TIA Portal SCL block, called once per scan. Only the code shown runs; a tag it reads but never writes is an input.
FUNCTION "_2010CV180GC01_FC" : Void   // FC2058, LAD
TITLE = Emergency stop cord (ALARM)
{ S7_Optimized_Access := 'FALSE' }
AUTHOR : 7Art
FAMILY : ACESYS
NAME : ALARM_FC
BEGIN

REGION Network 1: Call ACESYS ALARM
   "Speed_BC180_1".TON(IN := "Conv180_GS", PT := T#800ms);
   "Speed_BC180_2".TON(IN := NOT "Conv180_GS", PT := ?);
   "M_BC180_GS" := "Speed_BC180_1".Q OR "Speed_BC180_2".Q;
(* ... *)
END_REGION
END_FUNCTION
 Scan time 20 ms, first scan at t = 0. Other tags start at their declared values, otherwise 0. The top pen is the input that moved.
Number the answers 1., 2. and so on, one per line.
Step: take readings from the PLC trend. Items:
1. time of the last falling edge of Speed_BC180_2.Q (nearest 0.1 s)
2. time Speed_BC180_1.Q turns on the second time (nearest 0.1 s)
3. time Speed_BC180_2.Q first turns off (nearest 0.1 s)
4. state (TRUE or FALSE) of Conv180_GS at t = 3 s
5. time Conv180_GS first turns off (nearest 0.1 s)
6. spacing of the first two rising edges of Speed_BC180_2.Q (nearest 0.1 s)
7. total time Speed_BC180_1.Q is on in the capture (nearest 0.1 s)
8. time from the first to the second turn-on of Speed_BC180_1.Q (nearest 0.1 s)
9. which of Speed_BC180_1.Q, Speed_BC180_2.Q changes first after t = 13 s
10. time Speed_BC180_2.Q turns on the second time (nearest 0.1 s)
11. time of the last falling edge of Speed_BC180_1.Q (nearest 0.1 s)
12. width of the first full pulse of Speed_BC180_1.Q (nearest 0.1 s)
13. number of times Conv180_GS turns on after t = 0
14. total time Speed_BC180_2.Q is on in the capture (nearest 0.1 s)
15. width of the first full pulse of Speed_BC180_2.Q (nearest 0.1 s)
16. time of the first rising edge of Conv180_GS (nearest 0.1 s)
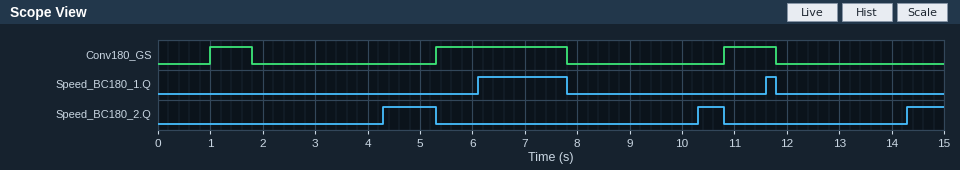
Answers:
1. 10.8 s
2. 11.6 s
3. 5.3 s
4. FALSE
5. 1.8 s
6. 6.0 s
7. 1.9 s
8. 5.5 s
9. Speed_BC180_2.Q
10. 10.3 s
11. 11.8 s
12. 1.7 s
13. 3
14. 2.2 s
15. 1.0 s
16. 1.0 s
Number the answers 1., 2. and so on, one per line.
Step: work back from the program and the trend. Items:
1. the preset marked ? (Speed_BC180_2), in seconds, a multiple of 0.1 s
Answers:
1. 2.5 s
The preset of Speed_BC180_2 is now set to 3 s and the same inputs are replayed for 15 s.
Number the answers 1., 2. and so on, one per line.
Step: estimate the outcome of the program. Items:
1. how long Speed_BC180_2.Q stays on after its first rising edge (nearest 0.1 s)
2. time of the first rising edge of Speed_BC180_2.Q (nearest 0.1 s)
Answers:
1. 0.5 s
2. 4.8 s
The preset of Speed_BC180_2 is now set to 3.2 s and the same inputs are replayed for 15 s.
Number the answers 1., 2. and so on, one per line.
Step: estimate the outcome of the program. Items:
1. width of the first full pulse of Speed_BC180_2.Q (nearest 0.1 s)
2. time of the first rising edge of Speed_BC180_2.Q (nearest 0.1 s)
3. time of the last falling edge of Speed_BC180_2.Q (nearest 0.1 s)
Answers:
1. 0.3 s
2. 5.0 s
3. 5.3 s
